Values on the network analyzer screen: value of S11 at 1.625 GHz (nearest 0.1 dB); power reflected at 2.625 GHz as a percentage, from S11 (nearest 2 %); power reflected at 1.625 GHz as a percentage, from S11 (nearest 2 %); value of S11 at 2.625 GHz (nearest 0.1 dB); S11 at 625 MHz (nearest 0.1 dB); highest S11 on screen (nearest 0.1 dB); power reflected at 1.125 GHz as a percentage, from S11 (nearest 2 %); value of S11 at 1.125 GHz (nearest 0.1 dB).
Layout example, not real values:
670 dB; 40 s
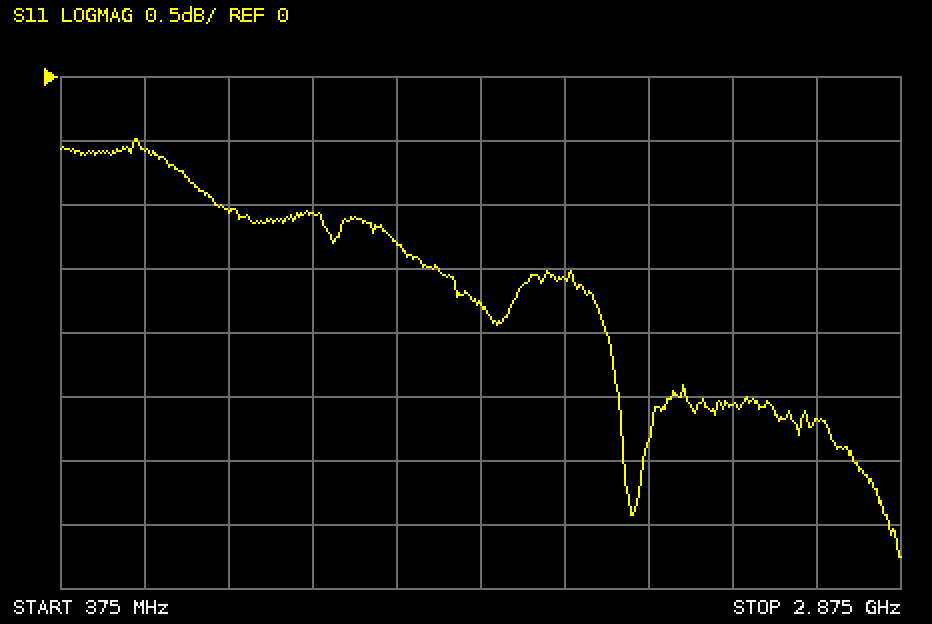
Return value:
-1.8 dB; 54 %; 66 %; -2.7 dB; -0.6 dB; -0.5 dB; 78 %; -1.1 dB
